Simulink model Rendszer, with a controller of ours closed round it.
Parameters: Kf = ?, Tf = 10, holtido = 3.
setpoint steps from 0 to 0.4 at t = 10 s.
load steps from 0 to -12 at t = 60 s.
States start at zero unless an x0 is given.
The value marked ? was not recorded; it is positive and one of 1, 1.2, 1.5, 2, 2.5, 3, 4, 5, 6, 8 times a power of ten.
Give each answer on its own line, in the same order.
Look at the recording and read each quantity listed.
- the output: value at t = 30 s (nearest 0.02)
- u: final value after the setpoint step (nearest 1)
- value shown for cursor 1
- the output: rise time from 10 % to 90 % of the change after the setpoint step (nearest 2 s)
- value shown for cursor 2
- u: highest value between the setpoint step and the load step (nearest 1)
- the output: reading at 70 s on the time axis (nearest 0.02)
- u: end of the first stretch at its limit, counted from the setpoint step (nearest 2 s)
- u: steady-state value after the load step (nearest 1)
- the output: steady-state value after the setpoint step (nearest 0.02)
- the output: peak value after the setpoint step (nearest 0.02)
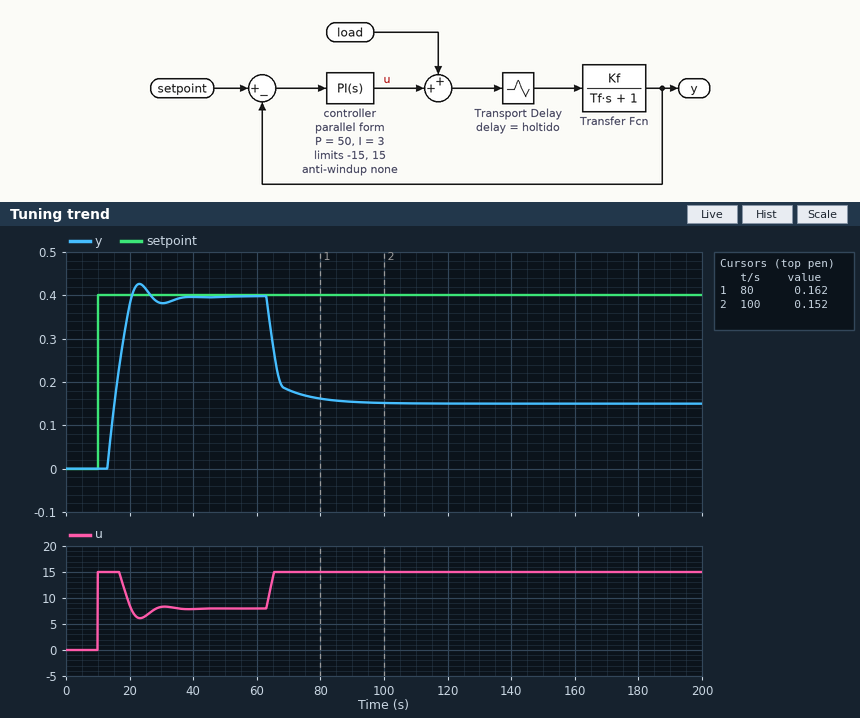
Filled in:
0.38
8
0.162
6 s
0.152
15
0.18
6 s
15
0.40
0.42
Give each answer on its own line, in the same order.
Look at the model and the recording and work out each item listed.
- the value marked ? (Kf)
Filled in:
0.05
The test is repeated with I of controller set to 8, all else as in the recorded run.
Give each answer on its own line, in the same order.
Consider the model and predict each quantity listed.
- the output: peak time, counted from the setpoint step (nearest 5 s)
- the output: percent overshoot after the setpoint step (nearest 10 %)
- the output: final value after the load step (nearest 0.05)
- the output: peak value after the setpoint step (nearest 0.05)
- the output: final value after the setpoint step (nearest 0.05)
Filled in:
20 s
40 %
0.15
0.55
0.40
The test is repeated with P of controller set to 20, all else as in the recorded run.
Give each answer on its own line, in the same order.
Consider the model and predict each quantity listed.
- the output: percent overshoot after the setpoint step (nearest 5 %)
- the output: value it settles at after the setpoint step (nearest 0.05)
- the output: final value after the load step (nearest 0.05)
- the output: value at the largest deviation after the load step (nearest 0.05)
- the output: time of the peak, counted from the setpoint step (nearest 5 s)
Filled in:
10 %
0.40
0.15
0.15
25 s
